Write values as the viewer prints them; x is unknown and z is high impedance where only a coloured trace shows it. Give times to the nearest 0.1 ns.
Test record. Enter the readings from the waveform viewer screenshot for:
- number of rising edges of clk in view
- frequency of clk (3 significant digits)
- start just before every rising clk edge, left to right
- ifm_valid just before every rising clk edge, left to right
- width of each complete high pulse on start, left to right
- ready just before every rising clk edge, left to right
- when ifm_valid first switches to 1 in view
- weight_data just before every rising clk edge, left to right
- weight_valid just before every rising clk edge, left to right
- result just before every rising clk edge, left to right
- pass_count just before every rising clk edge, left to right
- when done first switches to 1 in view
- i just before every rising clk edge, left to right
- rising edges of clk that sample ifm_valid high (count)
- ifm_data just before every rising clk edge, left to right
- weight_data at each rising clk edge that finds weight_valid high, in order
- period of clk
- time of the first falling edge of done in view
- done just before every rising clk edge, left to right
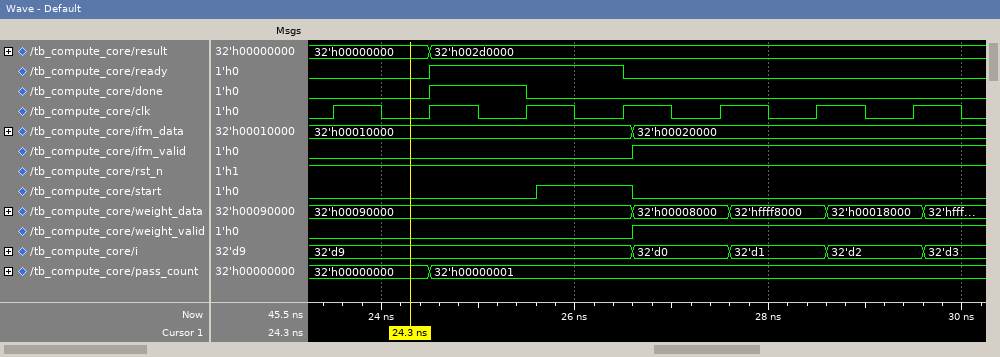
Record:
7
1.00 GHz
0 0 0 1 0 0 0
0 0 0 0 1 1 1
1 ns
0 0 1 1 0 0 0
26.6 ns
32'h00090000, 32'h00090000, 32'h00090000, 32'h00090000, 32'h00008000, 32'hffff8000, 32'h00018000
0 0 0 0 1 1 1
32'h00000000, 32'h00000000, 32'h002d0000, 32'h002d0000, 32'h002d0000, 32'h002d0000, 32'h002d0000
32'h00000000, 32'h00000000, 32'h00000001, 32'h00000001, 32'h00000001, 32'h00000001, 32'h00000001
24.5 ns
32'd9, 32'd9, 32'd9, 32'd9, 32'd0, 32'd1, 32'd2
3
32'h00010000, 32'h00010000, 32'h00010000, 32'h00010000, 32'h00020000, 32'h00020000, 32'h00020000
32'h00008000, 32'hffff8000, 32'h00018000
1 ns
25.5 ns
0 0 1 0 0 0 0
